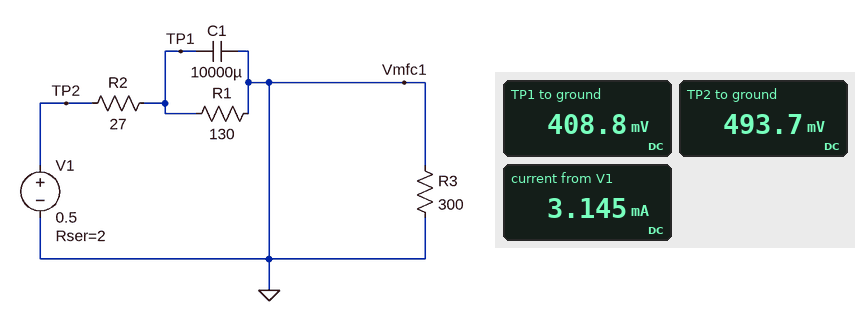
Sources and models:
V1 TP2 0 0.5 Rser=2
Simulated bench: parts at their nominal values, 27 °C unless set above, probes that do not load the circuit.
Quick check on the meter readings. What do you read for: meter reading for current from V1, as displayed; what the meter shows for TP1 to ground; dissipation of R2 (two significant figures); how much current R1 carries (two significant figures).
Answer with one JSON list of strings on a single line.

["3.145 mA", "408.8 mV", "270 µW", "3.1 mA"]
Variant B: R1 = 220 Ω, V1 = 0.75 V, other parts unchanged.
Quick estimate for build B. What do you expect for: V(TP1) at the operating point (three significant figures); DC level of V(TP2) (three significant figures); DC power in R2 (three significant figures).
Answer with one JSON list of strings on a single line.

["663 mV", "744 mV", "245 µW"]
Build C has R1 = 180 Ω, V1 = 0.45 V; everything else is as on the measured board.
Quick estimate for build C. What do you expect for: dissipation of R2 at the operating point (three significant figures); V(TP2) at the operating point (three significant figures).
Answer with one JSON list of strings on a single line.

["125 µW", "446 mV"]
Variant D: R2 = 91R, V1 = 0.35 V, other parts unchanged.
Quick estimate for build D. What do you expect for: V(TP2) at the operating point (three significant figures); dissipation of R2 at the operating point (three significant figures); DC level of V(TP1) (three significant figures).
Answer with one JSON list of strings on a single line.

["347 mV", "224 µW", "204 mV"]
